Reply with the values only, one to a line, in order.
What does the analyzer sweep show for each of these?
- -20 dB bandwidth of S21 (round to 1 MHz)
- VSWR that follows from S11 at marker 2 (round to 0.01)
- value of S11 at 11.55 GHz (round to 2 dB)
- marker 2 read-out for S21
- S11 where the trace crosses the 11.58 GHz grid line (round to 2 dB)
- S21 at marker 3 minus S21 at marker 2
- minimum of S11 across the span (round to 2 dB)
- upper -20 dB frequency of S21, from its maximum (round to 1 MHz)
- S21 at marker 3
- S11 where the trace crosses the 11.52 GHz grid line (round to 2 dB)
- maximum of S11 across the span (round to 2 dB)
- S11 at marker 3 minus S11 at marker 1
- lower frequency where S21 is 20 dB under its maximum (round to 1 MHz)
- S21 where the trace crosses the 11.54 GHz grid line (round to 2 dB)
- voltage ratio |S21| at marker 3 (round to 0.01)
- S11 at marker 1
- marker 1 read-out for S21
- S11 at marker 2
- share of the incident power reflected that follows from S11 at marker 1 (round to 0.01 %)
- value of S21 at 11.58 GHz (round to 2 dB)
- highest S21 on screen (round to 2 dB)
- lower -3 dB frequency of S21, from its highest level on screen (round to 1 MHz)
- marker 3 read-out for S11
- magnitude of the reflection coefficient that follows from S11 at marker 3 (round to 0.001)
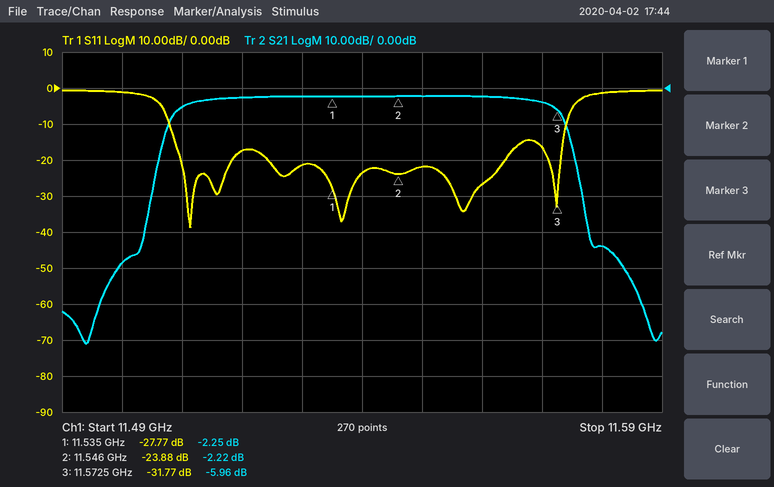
70 MHz
1.14
-22 dB
-2.22 dB
-2 dB
-3.74 dB
-38 dB
11.576 GHz
-5.96 dB
-18 dB
0 dB
-4.00 dB
11.506 GHz
-2 dB
0.50
-27.77 dB
-2.25 dB
-23.88 dB
0.17 %
-44 dB
-2 dB
11.510 GHz
-31.77 dB
0.026
